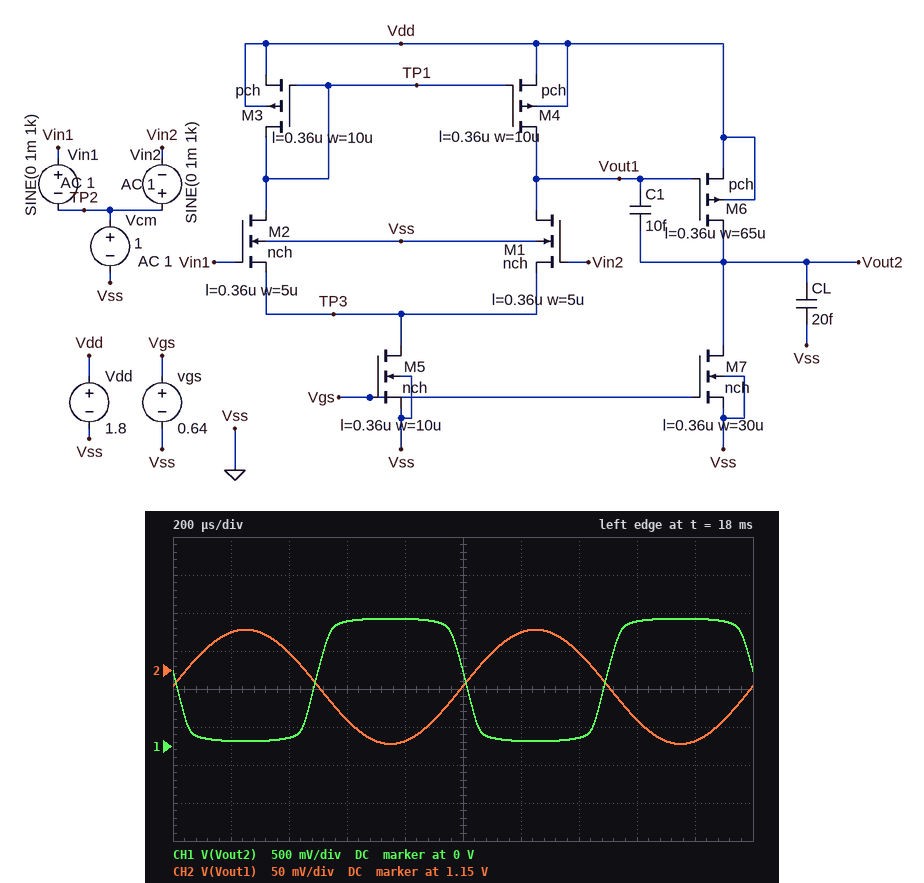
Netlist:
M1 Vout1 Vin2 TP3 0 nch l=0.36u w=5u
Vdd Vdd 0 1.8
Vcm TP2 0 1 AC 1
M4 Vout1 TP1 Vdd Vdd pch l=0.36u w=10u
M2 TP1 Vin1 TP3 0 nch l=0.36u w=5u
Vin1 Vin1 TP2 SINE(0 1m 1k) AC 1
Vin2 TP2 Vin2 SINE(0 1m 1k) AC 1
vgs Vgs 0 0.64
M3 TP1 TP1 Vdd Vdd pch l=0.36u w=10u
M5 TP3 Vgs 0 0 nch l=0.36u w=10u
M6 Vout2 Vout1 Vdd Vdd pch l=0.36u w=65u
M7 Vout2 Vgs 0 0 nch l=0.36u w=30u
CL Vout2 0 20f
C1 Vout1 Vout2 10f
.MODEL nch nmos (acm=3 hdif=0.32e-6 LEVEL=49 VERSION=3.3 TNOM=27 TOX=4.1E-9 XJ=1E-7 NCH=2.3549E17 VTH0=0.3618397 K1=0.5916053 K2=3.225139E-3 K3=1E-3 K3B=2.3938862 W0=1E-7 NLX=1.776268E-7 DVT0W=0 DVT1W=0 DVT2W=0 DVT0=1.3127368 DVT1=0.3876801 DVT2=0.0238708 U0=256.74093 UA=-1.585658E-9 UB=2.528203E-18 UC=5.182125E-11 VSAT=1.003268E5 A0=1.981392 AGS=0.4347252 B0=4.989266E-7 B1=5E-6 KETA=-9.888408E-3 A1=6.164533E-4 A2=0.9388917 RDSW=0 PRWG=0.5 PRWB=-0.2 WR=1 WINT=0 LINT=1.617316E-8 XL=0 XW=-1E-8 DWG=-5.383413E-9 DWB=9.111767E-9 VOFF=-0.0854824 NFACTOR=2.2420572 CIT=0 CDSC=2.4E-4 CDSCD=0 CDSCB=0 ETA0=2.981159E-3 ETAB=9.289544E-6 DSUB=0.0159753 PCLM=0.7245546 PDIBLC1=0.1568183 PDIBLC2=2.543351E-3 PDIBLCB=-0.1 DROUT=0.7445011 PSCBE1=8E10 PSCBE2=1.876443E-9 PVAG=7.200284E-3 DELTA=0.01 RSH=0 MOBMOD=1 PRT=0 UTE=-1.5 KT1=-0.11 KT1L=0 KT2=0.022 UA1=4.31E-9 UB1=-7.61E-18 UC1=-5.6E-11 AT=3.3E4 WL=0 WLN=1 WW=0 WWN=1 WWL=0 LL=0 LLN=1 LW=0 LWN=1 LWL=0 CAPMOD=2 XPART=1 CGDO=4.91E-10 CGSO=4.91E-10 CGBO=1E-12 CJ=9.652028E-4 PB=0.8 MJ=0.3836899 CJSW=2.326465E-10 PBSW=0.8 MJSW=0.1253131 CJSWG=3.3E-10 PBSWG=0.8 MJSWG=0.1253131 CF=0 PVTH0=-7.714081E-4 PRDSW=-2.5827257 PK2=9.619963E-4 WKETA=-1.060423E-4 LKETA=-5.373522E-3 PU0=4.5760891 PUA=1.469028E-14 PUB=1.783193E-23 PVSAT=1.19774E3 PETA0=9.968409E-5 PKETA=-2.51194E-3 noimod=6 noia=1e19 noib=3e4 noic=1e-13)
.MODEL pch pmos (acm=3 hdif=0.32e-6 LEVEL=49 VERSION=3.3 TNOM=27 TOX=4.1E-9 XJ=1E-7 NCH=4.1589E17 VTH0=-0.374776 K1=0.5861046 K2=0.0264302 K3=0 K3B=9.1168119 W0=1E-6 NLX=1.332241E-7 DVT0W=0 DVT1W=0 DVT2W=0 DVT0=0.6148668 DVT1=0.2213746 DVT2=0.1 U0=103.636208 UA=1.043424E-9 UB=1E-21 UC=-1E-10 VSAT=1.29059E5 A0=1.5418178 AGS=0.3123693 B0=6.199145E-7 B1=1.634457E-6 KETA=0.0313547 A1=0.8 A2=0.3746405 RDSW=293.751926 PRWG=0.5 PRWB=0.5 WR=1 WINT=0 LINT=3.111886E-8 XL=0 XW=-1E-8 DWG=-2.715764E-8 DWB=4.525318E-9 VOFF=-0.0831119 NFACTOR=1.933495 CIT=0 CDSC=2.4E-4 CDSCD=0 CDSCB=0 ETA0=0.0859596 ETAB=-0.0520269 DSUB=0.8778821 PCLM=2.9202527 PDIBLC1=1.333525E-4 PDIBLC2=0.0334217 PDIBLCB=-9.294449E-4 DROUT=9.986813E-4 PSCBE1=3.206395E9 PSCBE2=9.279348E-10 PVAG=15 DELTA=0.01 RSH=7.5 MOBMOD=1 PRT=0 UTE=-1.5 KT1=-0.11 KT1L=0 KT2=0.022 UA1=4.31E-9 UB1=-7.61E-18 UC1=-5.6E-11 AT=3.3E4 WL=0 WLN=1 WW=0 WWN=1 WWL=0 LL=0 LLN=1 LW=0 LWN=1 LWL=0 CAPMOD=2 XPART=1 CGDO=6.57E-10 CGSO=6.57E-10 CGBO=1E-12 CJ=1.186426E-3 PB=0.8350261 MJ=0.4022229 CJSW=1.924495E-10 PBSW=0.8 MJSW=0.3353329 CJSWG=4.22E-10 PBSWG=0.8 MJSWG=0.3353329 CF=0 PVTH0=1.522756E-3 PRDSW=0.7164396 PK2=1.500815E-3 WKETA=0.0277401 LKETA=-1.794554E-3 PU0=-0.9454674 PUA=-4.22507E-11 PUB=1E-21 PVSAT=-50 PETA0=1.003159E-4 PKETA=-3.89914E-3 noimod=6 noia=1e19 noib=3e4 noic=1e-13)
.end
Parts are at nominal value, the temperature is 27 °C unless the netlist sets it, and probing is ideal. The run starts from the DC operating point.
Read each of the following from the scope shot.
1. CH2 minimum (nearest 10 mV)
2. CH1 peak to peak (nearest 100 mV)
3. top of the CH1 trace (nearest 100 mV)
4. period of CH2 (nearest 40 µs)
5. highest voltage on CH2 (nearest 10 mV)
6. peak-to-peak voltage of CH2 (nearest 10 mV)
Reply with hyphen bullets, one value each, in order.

- 1.05 V
- 1.6 V
- 1.7 V
- 1.00 ms
- 1.20 V
- 150 mV
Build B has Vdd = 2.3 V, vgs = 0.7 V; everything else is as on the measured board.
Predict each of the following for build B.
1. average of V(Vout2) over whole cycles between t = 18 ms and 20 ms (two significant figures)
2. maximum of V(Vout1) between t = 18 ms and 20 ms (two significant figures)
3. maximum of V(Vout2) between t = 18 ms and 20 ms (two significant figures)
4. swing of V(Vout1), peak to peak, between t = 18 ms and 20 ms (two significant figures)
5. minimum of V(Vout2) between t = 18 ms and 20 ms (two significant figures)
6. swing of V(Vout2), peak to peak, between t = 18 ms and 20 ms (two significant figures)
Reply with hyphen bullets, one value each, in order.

- 1.1 V
- 1.6 V
- 2.1 V
- 140 mV
- 110 mV
- 2.0 V
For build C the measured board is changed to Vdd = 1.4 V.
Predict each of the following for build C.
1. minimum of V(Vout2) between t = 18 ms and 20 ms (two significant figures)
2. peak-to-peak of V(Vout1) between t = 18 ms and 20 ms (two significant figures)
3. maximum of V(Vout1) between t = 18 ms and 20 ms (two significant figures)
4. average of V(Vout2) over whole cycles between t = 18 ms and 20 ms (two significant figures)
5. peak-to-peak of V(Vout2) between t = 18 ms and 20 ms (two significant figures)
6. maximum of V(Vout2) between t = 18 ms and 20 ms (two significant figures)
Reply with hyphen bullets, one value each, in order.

- 64 mV
- 130 mV
- 800 mV
- 690 mV
- 1.2 V
- 1.3 V
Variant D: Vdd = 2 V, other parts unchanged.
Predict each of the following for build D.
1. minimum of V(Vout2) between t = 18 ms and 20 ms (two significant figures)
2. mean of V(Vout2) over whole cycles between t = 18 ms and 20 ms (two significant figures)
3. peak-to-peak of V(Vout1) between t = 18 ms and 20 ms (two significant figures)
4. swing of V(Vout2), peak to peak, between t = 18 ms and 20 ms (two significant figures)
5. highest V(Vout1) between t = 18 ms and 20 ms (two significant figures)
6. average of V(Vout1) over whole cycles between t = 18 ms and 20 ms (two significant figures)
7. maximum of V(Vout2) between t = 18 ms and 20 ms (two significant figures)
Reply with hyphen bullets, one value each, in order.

- 62 mV
- 990 mV
- 150 mV
- 1.8 V
- 1.4 V
- 1.3 V
- 1.9 V
